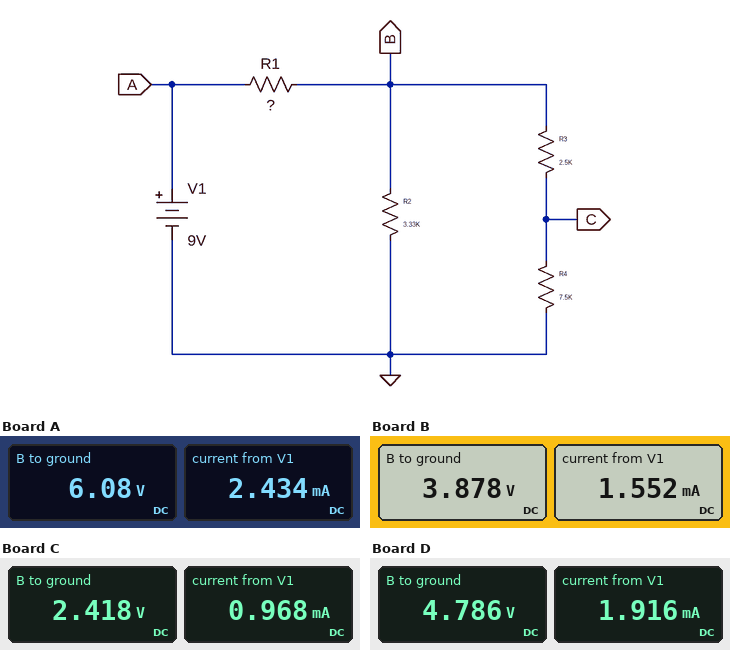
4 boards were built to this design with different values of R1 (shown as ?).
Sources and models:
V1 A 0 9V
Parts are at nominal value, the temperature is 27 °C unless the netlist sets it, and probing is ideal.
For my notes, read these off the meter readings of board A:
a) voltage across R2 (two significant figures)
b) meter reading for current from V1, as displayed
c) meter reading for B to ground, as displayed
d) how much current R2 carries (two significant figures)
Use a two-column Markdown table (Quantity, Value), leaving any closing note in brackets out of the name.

| Quantity | Value |
|---|---|
| voltage across R2 | 6.1 V |
| meter reading for current from V1, as displayed | 2.434 mA |
| meter reading for B to ground, as displayed | 6.08 V |
| how much current R2 carries | 1.8 mA |
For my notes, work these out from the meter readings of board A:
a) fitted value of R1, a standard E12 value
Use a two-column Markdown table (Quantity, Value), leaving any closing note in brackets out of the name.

| Quantity | Value |
|---|---|
| fitted value of R1, a standard E12 value | 1.2 kΩ |
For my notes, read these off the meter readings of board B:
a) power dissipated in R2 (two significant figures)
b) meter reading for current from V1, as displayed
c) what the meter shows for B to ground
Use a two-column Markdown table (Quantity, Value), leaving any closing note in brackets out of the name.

| Quantity | Value |
|---|---|
| power dissipated in R2 | 4.5 mW |
| meter reading for current from V1, as displayed | 1.552 mA |
| what the meter shows for B to ground | 3.878 V |
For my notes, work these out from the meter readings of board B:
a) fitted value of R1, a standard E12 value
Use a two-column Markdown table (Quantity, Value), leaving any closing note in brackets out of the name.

| Quantity | Value |
|---|---|
| fitted value of R1, a standard E12 value | 3.3 kΩ |
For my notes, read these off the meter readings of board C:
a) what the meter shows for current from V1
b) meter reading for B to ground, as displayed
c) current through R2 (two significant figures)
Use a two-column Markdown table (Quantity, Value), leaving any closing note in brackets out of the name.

| Quantity | Value |
|---|---|
| what the meter shows for current from V1 | 0.968 mA |
| meter reading for B to ground, as displayed | 2.418 V |
| current through R2 | 730 µA |
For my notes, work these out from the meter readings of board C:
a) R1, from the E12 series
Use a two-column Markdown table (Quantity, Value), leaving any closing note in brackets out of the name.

| Quantity | Value |
|---|---|
| R1, from the E12 series | 6.8 kΩ |
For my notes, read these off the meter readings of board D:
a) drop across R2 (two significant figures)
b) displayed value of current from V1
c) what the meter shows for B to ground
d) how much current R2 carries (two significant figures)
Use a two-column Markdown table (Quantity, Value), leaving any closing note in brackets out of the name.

| Quantity | Value |
|---|---|
| drop across R2 | 4.8 V |
| displayed value of current from V1 | 1.916 mA |
| what the meter shows for B to ground | 4.786 V |
| how much current R2 carries | 1.4 mA |
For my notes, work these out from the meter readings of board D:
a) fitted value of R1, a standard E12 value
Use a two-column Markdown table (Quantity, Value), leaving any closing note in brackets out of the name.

| Quantity | Value |
|---|---|
| fitted value of R1, a standard E12 value | 2.2 kΩ |
